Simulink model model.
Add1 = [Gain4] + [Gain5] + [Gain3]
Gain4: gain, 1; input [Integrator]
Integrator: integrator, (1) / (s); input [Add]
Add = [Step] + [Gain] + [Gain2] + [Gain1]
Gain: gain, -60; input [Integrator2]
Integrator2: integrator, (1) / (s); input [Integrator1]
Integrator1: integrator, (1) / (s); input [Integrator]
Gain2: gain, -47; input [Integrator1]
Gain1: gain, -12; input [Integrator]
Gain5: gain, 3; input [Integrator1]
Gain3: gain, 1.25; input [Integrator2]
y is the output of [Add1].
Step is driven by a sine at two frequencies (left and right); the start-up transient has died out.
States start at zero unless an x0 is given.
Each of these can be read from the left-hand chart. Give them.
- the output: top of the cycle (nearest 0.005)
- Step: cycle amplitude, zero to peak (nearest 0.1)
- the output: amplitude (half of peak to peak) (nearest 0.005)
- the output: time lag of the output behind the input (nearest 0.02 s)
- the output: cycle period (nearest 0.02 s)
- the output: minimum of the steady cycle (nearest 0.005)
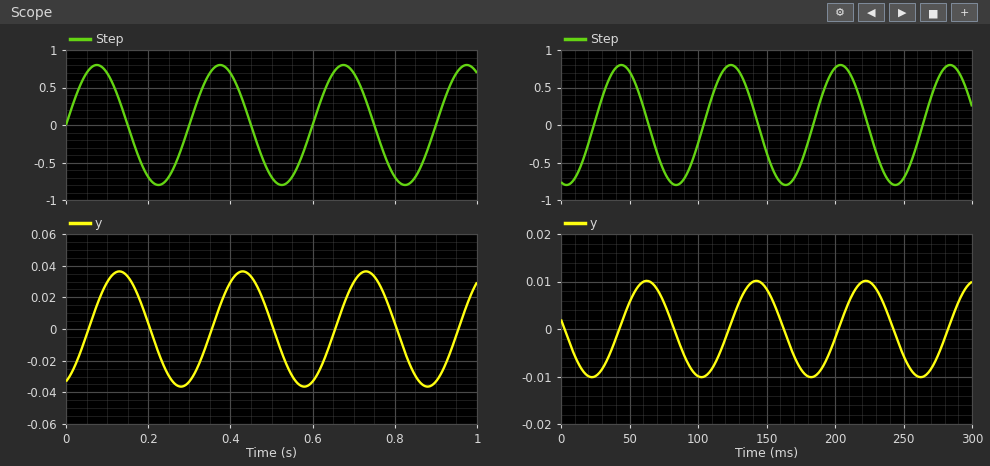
0.035
0.8
0.035
0.06 s
0.30 s
-0.035
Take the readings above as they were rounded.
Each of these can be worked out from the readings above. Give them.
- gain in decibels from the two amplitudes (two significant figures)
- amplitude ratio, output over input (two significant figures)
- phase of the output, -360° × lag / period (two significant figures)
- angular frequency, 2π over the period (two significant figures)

-27 dB
0.044
-72°
21 rad/s
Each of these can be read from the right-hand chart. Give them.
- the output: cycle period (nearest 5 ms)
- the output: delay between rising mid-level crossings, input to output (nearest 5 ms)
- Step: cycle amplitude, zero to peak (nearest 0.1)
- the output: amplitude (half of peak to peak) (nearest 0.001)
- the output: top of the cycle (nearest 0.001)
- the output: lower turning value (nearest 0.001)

80 ms
20 ms
0.8
0.010
0.010
-0.010
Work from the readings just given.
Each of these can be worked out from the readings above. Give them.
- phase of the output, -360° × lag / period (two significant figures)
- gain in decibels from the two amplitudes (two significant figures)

-90°
-38 dB
